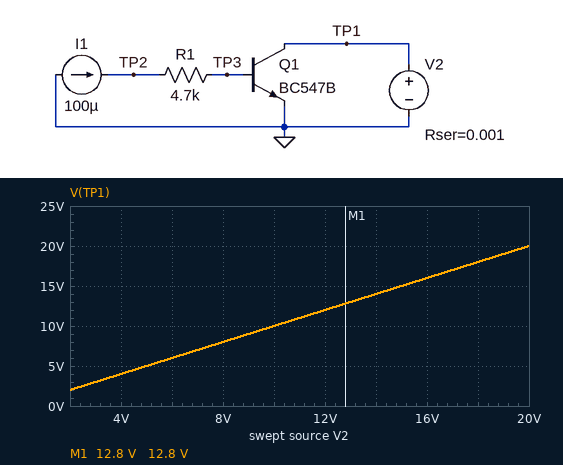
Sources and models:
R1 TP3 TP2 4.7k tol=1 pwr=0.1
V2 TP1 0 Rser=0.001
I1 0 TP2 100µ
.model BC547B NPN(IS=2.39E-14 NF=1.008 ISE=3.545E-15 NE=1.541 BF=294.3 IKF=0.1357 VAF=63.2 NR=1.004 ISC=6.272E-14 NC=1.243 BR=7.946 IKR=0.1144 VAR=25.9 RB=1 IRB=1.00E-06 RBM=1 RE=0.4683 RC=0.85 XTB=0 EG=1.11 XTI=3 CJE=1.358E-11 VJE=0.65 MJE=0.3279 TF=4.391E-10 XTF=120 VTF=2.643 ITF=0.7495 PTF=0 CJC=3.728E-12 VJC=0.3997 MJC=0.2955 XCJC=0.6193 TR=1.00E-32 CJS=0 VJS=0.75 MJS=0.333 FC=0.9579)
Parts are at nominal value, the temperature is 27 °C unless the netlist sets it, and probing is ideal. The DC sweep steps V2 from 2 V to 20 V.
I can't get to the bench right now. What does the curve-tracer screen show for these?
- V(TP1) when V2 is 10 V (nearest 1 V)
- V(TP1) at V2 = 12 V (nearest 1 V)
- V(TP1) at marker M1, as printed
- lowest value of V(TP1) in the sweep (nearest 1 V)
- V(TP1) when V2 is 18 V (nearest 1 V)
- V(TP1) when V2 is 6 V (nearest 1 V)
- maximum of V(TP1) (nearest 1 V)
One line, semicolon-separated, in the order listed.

10 V; 12 V; 12.8 V; 2 V; 18 V; 6 V; 20 V
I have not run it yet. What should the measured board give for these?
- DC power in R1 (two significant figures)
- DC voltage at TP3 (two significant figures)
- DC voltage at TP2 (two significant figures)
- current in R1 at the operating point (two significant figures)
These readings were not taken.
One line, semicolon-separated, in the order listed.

47 µW; 620 mV; 1.1 V; 100 µA
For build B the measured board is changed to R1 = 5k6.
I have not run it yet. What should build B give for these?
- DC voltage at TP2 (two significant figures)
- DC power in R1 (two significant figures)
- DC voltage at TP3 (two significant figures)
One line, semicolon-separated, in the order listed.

1.2 V; 56 µW; 620 mV
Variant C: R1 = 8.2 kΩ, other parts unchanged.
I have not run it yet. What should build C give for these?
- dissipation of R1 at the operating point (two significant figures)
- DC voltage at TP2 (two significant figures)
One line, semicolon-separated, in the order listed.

82 µW; 1.4 V
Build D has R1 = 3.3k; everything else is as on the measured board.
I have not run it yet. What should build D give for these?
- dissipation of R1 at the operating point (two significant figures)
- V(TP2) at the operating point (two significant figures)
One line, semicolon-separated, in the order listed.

33 µW; 950 mV
